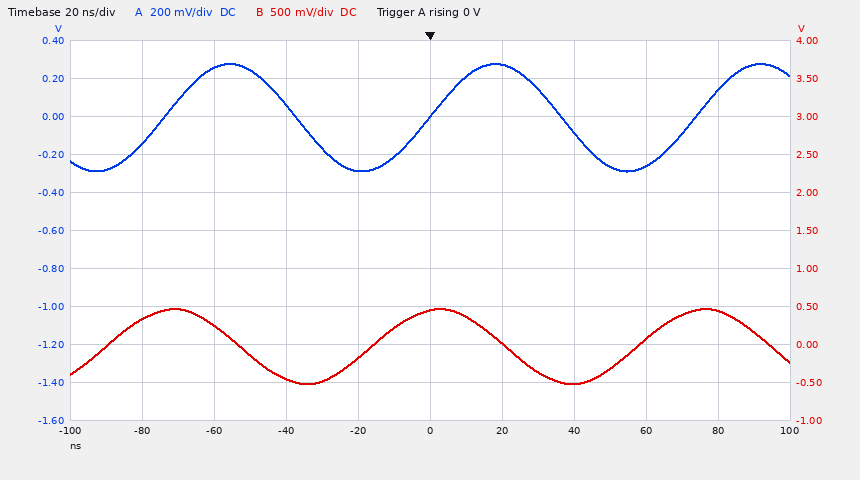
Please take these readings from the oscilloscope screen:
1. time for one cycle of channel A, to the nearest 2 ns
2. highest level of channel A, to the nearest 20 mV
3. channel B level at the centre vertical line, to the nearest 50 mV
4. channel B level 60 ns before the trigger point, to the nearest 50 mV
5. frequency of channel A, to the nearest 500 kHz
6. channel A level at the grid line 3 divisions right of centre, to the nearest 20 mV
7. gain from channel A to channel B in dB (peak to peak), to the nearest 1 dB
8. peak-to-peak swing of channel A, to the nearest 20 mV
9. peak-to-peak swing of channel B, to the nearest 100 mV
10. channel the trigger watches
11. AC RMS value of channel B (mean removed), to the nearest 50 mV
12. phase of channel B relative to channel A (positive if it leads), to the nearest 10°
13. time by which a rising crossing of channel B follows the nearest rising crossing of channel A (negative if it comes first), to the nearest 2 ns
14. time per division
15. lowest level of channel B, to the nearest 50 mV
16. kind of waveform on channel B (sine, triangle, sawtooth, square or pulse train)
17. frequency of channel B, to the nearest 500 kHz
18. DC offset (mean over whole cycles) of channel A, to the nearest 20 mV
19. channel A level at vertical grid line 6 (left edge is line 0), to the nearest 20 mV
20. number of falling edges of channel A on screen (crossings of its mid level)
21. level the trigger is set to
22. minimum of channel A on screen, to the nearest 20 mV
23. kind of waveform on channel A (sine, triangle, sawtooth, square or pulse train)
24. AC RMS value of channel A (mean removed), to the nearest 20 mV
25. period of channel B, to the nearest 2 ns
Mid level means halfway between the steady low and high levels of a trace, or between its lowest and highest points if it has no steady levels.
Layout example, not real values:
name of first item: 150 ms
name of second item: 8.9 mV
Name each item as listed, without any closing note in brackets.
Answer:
time for one cycle of channel A, to the nearest 2 ns: 74 ns
highest level of channel A, to the nearest 20 mV: 280 mV
channel B level at the centre vertical line, to the nearest 50 mV: 450 mV
channel B level 60 ns before the trigger point, to the nearest 50 mV: 250 mV
frequency of channel A, to the nearest 500 kHz: 13.5 MHz
channel A level at the grid line 3 divisions right of centre, to the nearest 20 mV: -260 mV
gain from channel A to channel B in dB (peak to peak), to the nearest 1 dB: 5 dB
peak-to-peak swing of channel A, to the nearest 20 mV: 560 mV
peak-to-peak swing of channel B, to the nearest 100 mV: 1.00 V
channel the trigger watches: channel A
AC RMS value of channel B (mean removed), to the nearest 50 mV: 350 mV
phase of channel B relative to channel A (positive if it leads), to the nearest 10°: +80°
time by which a rising crossing of channel B follows the nearest rising crossing of channel A (negative if it comes first), to the nearest 2 ns: -16 ns
time per division: 20 ns
lowest level of channel B, to the nearest 50 mV: -500 mV
kind of waveform on channel B: sine
frequency of channel B, to the nearest 500 kHz: 13.5 MHz
DC offset (mean over whole cycles) of channel A, to the nearest 20 mV: 0 mV
channel A level at vertical grid line 6 (left edge is line 0), to the nearest 20 mV: 280 mV
number of falling edges of channel A on screen: 2
level the trigger is set to: 0 V
minimum of channel A on screen, to the nearest 20 mV: -280 mV
kind of waveform on channel A: sine
AC RMS value of channel A (mean removed), to the nearest 20 mV: 200 mV
period of channel B, to the nearest 2 ns: 74 ns
